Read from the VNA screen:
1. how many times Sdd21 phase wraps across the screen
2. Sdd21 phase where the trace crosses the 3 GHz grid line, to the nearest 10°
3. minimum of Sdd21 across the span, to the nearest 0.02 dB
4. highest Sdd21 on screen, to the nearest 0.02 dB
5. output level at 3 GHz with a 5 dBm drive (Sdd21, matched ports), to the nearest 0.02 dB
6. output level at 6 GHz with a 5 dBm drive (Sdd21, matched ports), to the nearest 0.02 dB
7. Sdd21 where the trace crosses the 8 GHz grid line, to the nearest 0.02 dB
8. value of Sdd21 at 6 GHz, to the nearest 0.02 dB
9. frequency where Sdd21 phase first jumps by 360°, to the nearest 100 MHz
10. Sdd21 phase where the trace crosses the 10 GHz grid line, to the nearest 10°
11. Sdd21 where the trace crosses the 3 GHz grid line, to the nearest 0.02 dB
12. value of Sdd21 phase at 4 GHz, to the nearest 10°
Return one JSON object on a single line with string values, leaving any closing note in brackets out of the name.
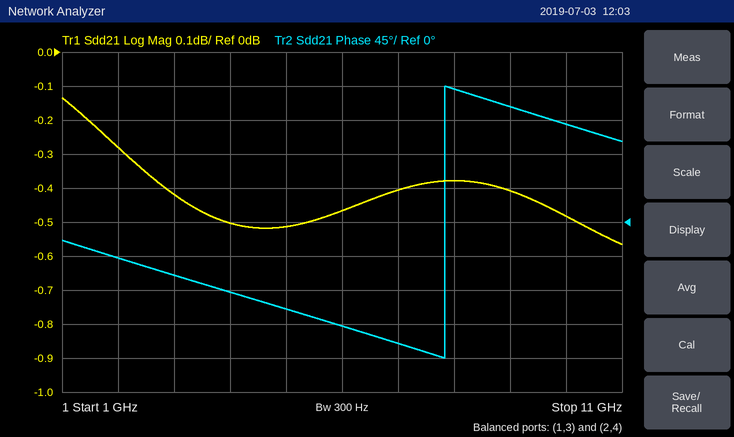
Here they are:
{"how many times Sdd21 phase wraps across the screen": "1", "Sdd21 phase where the trace crosses the 3 GHz grid line, to the nearest 10°": "-70°", "minimum of Sdd21 across the span, to the nearest 0.02 dB": "-0.56 dB", "highest Sdd21 on screen, to the nearest 0.02 dB": "-0.14 dB", "output level at 3 GHz with a 5 dBm drive (Sdd21, matched ports), to the nearest 0.02 dB": "4.58 dBm", "output level at 6 GHz with a 5 dBm drive (Sdd21, matched ports), to the nearest 0.02 dB": "4.54 dBm", "Sdd21 where the trace crosses the 8 GHz grid line, to the nearest 0.02 dB": "-0.38 dB", "value of Sdd21 at 6 GHz, to the nearest 0.02 dB": "-0.46 dB", "frequency where Sdd21 phase first jumps by 360°, to the nearest 100 MHz": "7.8 GHz", "Sdd21 phase where the trace crosses the 10 GHz grid line, to the nearest 10°": "130°", "Sdd21 where the trace crosses the 3 GHz grid line, to the nearest 0.02 dB": "-0.42 dB", "value of Sdd21 phase at 4 GHz, to the nearest 10°": "-90°"}
